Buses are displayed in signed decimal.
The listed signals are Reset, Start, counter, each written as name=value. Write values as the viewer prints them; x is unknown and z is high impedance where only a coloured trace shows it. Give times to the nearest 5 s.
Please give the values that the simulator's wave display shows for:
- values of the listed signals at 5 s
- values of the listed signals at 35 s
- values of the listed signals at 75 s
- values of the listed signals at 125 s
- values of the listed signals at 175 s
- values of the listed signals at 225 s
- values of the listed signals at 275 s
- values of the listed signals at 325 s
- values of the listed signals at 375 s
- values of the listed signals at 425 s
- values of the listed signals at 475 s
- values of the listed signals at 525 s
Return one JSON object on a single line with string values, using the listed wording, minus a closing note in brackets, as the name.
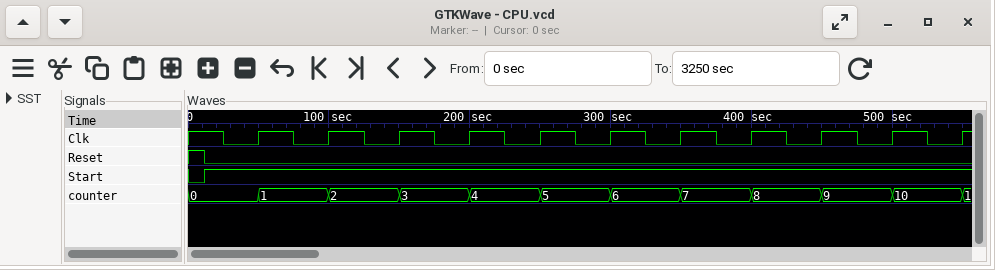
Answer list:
{"values of the listed signals at 5 s": "Reset=1, Start=0, counter=0", "values of the listed signals at 35 s": "Reset=0, Start=1, counter=0", "values of the listed signals at 75 s": "Reset=0, Start=1, counter=1", "values of the listed signals at 125 s": "Reset=0, Start=1, counter=2", "values of the listed signals at 175 s": "Reset=0, Start=1, counter=3", "values of the listed signals at 225 s": "Reset=0, Start=1, counter=4", "values of the listed signals at 275 s": "Reset=0, Start=1, counter=5", "values of the listed signals at 325 s": "Reset=0, Start=1, counter=6", "values of the listed signals at 375 s": "Reset=0, Start=1, counter=7", "values of the listed signals at 425 s": "Reset=0, Start=1, counter=8", "values of the listed signals at 475 s": "Reset=0, Start=1, counter=9", "values of the listed signals at 525 s": "Reset=0, Start=1, counter=10"}
